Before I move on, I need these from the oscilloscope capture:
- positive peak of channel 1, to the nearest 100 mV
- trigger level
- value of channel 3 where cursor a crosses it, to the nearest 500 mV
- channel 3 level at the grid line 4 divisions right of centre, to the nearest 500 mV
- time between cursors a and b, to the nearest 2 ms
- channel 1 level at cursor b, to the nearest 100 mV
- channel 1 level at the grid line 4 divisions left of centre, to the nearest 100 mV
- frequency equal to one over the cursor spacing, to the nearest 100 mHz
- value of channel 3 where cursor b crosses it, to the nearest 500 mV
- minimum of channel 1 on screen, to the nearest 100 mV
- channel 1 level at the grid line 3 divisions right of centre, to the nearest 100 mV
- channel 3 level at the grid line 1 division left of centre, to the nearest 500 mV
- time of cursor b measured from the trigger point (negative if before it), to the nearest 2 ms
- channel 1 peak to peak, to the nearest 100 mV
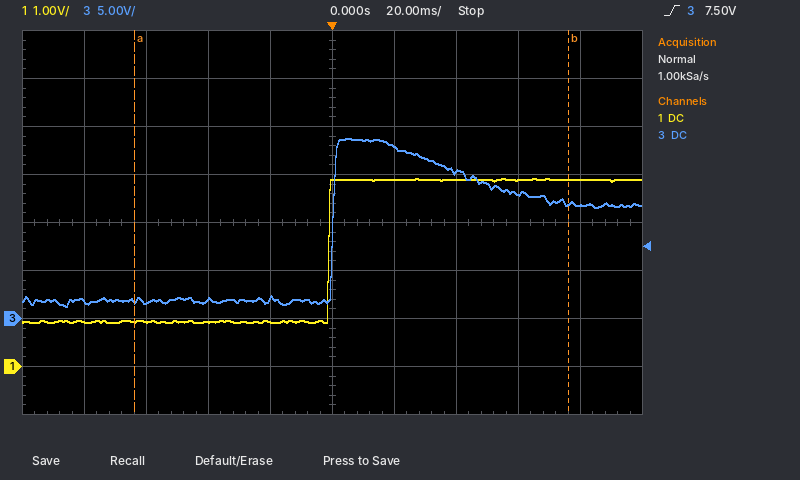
3.9 V
7.50 V
2.0 V
12.0 V
140 ms
3.9 V
900 mV
7.1 Hz
12.0 V
900 mV
3.9 V
2.0 V
+76 ms
3.0 V
